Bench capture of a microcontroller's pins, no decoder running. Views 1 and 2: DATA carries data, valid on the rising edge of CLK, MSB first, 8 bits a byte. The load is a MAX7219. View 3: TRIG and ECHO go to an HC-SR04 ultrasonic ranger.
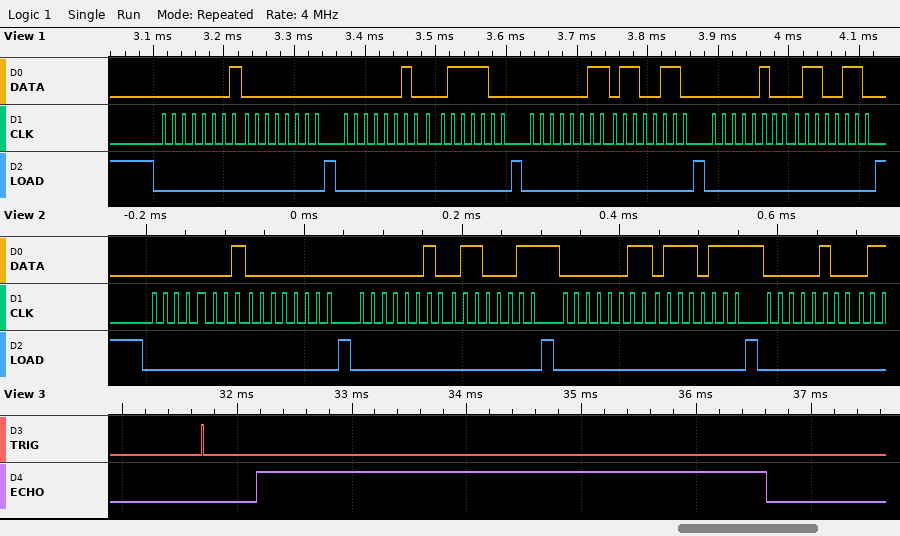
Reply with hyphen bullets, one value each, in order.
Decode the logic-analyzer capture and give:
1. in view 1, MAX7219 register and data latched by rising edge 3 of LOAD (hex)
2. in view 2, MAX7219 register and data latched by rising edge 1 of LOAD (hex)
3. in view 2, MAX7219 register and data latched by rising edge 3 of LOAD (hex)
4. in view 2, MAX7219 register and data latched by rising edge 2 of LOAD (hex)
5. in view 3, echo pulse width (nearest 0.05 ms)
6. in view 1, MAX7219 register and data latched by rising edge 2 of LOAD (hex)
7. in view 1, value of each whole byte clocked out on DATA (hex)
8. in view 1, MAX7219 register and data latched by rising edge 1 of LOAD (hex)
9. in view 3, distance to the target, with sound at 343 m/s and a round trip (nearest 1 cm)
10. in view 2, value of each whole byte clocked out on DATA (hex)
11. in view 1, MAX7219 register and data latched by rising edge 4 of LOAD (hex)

- register 0x3, data 0x66
- register 0x1, data 0x00
- register 0x3, data 0x77
- register 0x2, data 0x63
- 4.45 ms
- register 0x2, data 0x3C
- 01 00 02 3C 03 66 04 66
- register 0x1, data 0x00
- 76 cm
- 01 00 02 63 03 77 04
- register 0x4, data 0x66
